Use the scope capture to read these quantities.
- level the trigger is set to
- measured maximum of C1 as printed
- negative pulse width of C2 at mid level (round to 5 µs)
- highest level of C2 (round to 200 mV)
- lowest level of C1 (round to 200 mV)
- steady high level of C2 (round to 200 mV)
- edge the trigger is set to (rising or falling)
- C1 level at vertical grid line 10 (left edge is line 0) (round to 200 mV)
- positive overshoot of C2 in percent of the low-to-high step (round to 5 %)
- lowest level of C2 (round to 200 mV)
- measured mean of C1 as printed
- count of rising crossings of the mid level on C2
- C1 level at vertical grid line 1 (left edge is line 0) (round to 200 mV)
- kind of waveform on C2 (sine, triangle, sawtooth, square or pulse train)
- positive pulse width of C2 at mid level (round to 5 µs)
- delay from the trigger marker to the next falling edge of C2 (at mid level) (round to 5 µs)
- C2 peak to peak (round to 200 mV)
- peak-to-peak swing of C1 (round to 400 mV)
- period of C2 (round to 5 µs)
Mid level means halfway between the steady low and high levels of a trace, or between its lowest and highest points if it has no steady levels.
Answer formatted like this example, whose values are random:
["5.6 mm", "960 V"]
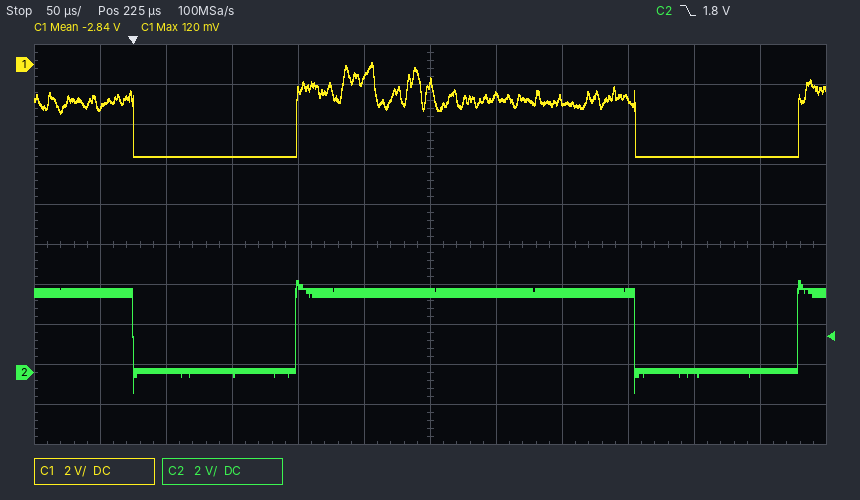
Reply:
["1.8 V", "120 mV", "125 µs", "4.6 V", "-4.6 V", "4.0 V", "falling", "-4.6 V", "15 %", "-1.0 V", "-2.84 V", "2", "-2.2 V", "pulse train", "255 µs", "380 µs", "5.6 V", "4.8 V", "380 µs"]
